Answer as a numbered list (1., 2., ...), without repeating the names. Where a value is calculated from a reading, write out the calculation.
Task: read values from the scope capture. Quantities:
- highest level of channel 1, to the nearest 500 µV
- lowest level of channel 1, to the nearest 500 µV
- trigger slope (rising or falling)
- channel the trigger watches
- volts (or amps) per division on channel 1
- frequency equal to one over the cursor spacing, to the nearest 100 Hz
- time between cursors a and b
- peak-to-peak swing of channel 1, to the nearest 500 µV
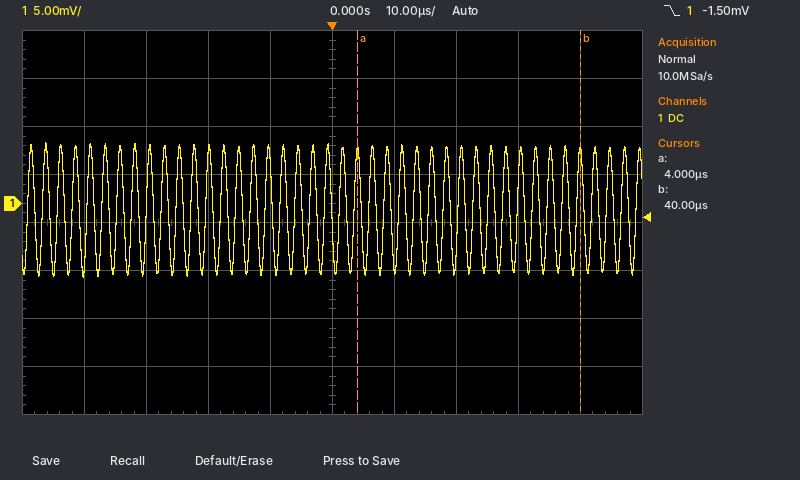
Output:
1. 6.5 mV
2. -7.5 mV
3. falling
4. channel 1
5. 5 mV
6. 1 / 36 µs ≈ 27.8 kHz
7. 40 µs − (4 µs) = 36 µs
8. 6.5 mV − (-7.5 mV) = 14.0 mV
